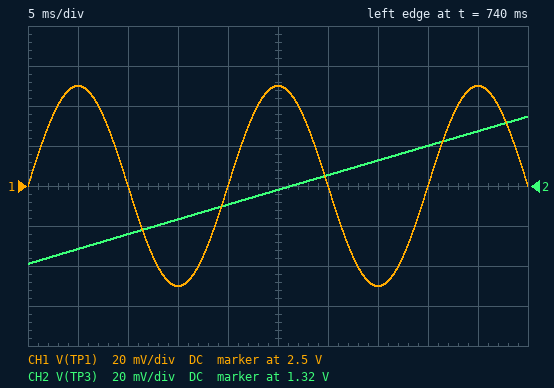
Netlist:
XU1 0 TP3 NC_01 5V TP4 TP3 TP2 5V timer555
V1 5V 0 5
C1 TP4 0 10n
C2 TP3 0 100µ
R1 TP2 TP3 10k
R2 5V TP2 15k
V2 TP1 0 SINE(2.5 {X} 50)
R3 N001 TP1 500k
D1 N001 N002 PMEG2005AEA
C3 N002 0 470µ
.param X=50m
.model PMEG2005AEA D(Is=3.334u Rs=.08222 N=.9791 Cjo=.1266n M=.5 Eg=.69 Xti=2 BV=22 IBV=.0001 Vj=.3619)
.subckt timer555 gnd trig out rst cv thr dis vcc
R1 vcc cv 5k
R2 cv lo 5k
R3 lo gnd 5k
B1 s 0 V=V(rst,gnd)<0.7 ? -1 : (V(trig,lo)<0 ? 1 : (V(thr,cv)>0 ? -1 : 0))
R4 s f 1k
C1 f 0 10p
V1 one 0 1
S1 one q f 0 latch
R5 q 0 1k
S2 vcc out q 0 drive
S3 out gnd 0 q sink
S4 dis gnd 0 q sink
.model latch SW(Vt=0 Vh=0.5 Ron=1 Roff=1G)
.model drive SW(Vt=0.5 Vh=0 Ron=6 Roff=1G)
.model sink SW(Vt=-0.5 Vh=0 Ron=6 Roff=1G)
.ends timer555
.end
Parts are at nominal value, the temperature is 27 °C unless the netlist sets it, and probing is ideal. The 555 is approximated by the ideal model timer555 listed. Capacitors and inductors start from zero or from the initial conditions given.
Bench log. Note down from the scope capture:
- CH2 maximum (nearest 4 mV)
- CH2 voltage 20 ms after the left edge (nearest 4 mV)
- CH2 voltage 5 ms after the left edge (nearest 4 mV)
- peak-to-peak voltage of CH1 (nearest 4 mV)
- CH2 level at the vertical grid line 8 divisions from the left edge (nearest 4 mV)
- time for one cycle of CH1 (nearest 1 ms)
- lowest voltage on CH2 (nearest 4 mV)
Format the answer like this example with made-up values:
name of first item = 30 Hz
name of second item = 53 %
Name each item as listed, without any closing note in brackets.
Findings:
CH2 maximum = 1.356 V
CH2 voltage 20 ms after the left edge = 1.312 V
CH2 voltage 5 ms after the left edge = 1.288 V
peak-to-peak voltage of CH1 = 100 mV
CH2 level at the vertical grid line 8 divisions from the left edge = 1.340 V
time for one cycle of CH1 = 20 ms
lowest voltage on CH2 = 1.280 V
